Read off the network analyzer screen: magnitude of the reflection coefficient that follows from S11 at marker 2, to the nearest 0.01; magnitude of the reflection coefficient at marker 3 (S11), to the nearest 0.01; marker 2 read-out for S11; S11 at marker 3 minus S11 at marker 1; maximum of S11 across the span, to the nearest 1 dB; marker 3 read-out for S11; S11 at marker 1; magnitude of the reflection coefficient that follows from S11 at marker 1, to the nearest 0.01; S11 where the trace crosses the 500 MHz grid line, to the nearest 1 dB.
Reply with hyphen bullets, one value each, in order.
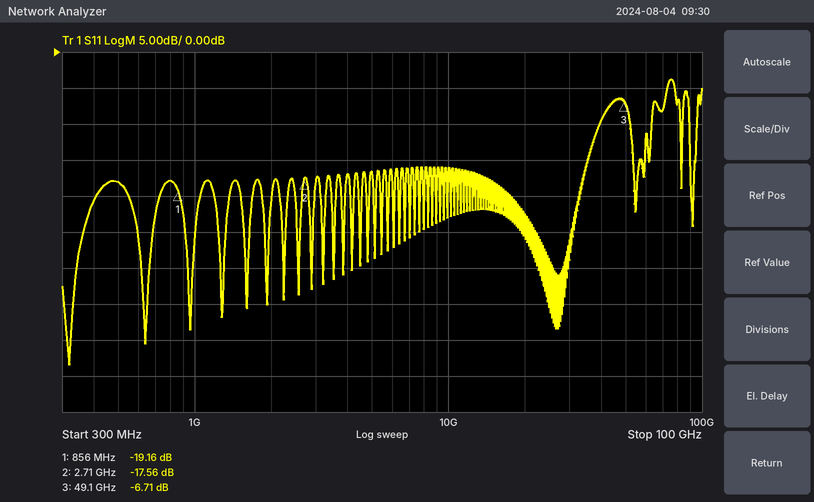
- 0.13
- 0.46
- -17.56 dB
- 12.45 dB
- -4 dB
- -6.71 dB
- -19.16 dB
- 0.11
- -18 dB
